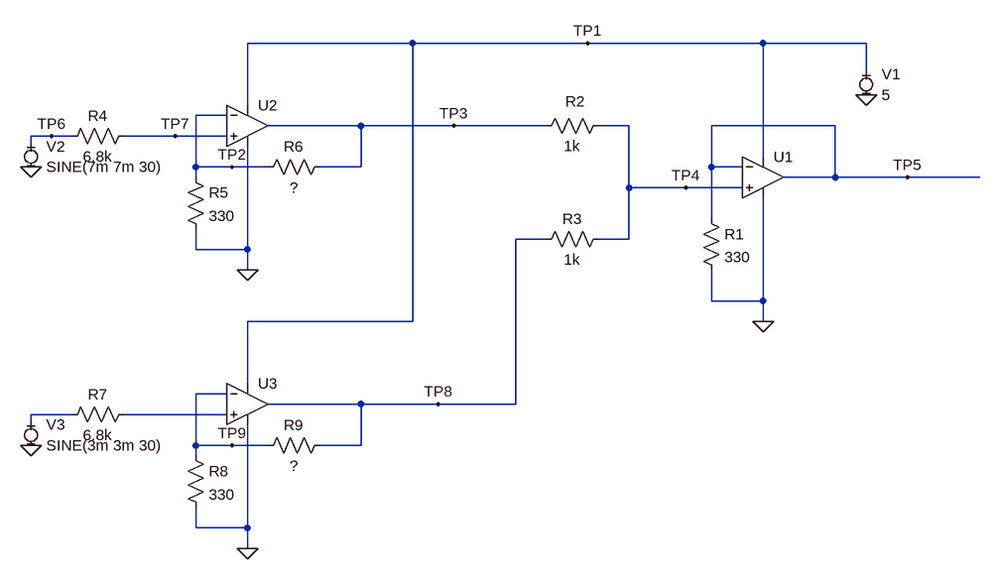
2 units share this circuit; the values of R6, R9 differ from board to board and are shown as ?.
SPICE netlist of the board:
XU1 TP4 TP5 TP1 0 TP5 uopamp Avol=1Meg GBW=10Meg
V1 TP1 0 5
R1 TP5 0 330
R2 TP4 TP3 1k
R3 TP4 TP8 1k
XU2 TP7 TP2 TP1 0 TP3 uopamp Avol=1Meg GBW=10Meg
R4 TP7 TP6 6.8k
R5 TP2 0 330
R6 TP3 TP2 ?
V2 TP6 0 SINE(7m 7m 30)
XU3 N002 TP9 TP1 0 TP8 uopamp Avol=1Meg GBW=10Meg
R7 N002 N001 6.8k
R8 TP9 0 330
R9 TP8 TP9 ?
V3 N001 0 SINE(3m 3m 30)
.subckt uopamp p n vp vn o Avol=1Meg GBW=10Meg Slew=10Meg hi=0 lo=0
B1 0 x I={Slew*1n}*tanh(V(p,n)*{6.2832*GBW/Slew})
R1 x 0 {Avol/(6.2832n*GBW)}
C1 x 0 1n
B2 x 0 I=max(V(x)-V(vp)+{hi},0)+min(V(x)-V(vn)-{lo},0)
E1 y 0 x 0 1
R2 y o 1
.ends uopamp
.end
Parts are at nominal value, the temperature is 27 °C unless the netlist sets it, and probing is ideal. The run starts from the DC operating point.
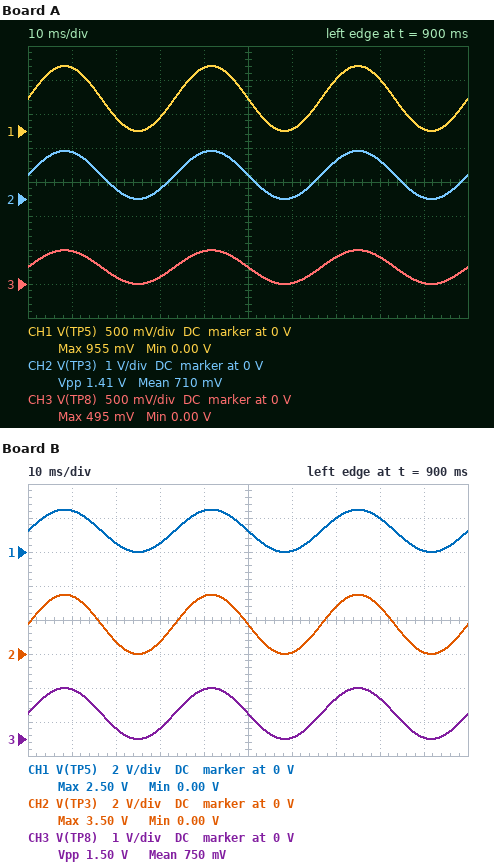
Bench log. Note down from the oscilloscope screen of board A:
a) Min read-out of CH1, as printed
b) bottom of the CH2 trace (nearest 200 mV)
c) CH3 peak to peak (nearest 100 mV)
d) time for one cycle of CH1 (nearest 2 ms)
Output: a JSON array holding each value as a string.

["0.00 V", "0 V", "500 mV", "34 ms"]
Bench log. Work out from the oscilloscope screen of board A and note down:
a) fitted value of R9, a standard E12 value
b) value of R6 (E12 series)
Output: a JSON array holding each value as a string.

["27 kΩ", "33 kΩ"]
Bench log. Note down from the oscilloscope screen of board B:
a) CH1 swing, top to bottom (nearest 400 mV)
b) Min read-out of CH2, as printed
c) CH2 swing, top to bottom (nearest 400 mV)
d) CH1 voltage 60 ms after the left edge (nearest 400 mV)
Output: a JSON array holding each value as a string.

["2.4 V", "0.00 V", "3.6 V", "0 V"]
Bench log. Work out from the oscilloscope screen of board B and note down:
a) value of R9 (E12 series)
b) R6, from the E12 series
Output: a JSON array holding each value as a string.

["82 kΩ", "82 kΩ"]
